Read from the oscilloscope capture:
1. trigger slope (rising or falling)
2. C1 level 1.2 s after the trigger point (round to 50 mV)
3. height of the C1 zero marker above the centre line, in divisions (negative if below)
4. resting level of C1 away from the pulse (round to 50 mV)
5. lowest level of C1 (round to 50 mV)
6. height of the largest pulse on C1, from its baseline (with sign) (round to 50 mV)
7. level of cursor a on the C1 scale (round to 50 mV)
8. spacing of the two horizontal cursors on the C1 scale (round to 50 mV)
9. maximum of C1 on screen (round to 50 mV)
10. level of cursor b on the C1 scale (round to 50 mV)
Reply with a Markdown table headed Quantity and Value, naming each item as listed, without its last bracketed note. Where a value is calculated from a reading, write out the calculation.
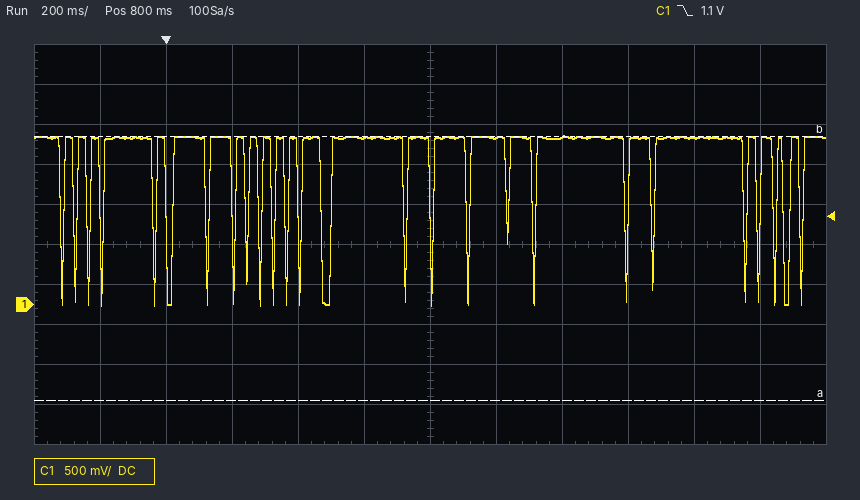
| Quantity | Value |
|---|---|
| trigger slope | falling |
| C1 level 1.2 s after the trigger point | 2.10 V |
| height of the C1 zero marker above the centre line, in divisions | -1.5 div |
| resting level of C1 away from the pulse | 2.10 V |
| lowest level of C1 | 0 mV |
| height of the largest pulse on C1, from its baseline (with sign) | 0 mV − (2.10 V) = -2.10 V |
| level of cursor a on the C1 scale | -1.20 V |
| spacing of the two horizontal cursors on the C1 scale | 3.30 V |
| maximum of C1 on screen | 2.10 V |
| level of cursor b on the C1 scale | 2.10 V |
